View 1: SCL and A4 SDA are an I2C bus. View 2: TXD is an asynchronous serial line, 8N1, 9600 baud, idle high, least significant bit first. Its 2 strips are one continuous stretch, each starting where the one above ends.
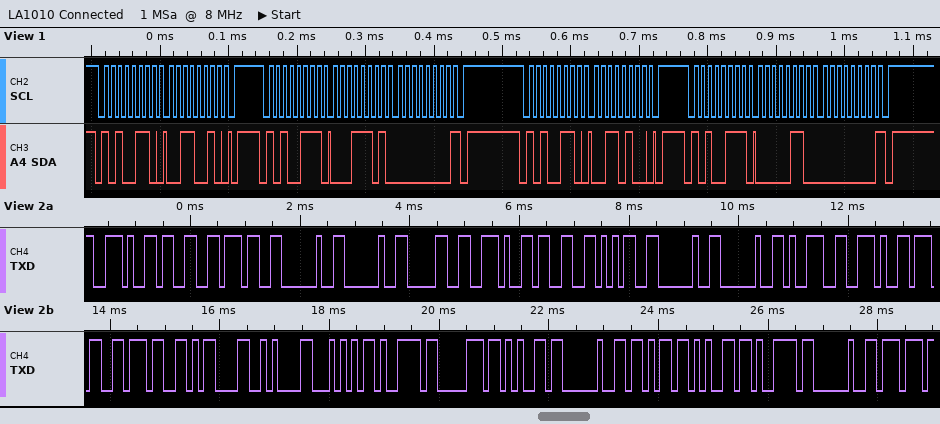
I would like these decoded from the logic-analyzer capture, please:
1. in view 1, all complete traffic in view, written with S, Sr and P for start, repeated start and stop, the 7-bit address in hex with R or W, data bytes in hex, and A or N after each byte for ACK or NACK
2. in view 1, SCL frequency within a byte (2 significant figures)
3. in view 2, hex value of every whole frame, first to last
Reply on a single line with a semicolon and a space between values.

S 53W A 32 A P S 53R A 1D A 00 N P S 53W A 34 A P S 53R A 06 A 00 N P; 100 kHz; 2E 33 37 20 20 30 2E 33 35 20 20 39 2E 37 37 0D 0A 54 79 70 65 20 6B 65 79 20 77
